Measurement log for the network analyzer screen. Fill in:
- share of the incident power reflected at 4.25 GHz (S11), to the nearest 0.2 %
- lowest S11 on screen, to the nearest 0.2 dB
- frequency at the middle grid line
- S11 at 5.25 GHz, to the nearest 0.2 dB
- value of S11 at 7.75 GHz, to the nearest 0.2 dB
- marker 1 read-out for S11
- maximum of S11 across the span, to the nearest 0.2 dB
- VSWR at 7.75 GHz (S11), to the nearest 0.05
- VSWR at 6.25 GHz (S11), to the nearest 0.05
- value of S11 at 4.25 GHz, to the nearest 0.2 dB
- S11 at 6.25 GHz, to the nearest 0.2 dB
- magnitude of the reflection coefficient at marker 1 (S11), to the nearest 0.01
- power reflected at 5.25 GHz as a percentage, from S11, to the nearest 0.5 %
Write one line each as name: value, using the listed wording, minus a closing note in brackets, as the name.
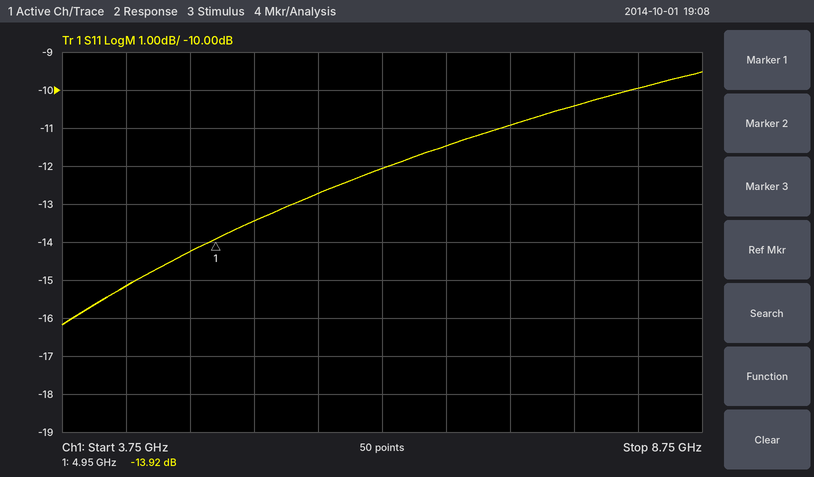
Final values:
share of the incident power reflected at 4.25 GHz (S11), to the nearest 0.2 %: 3.0 %
lowest S11 on screen, to the nearest 0.2 dB: -16.2 dB
frequency at the middle grid line: 6.25 GHz
S11 at 5.25 GHz, to the nearest 0.2 dB: -13.4 dB
value of S11 at 7.75 GHz, to the nearest 0.2 dB: -10.4 dB
marker 1 read-out for S11: -13.92 dB
maximum of S11 across the span, to the nearest 0.2 dB: -9.6 dB
VSWR at 7.75 GHz (S11), to the nearest 0.05: 1.85
VSWR at 6.25 GHz (S11), to the nearest 0.05: 1.65
value of S11 at 4.25 GHz, to the nearest 0.2 dB: -15.2 dB
S11 at 6.25 GHz, to the nearest 0.2 dB: -12.0 dB
magnitude of the reflection coefficient at marker 1 (S11), to the nearest 0.01: 0.20
power reflected at 5.25 GHz as a percentage, from S11, to the nearest 0.5 %: 4.5 %
